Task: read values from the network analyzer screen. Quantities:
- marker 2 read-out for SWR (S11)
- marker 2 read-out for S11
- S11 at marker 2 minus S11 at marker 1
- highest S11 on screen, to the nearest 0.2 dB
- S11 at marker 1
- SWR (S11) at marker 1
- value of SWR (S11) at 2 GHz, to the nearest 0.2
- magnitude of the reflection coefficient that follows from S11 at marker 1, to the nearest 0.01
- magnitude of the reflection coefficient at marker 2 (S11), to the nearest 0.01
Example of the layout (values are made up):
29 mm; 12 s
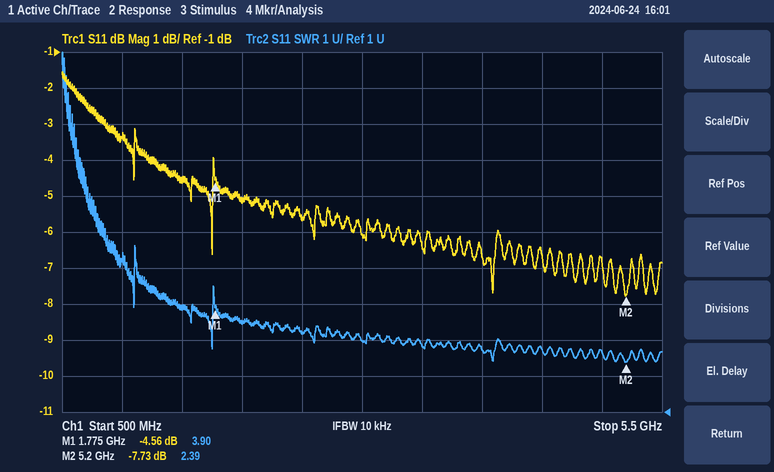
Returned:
2.39; -7.73 dB; -3.17 dB; -1.6 dB; -4.56 dB; 3.90; 3.4; 0.59; 0.41
